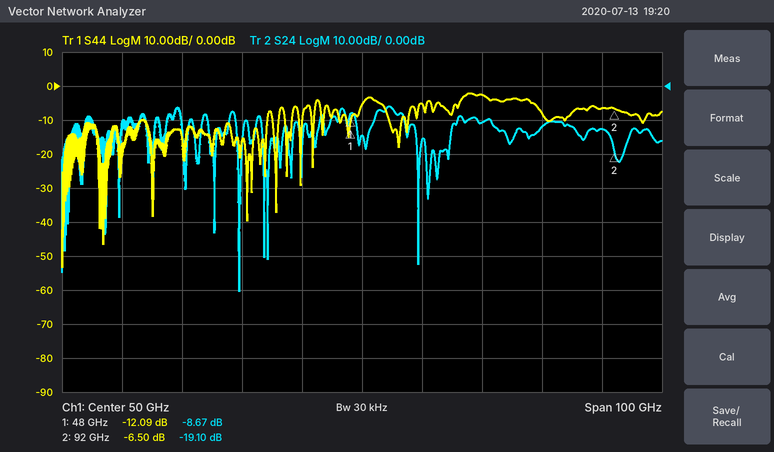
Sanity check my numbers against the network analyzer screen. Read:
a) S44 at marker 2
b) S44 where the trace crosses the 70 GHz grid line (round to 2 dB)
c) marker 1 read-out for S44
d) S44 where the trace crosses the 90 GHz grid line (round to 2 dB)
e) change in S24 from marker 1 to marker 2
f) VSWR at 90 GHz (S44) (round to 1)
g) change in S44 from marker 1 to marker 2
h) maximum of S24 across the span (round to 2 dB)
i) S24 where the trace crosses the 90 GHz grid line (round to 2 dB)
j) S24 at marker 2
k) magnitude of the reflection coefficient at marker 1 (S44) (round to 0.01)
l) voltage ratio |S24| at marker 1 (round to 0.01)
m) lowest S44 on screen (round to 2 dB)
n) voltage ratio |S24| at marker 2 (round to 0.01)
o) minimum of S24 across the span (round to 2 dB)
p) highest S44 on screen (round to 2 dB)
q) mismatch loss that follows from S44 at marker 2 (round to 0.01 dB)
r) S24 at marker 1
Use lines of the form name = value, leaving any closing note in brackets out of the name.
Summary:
S44 at marker 2 = -6.50 dB
S44 where the trace crosses the 70 GHz grid line = -2 dB
marker 1 read-out for S44 = -12.09 dB
S44 where the trace crosses the 90 GHz grid line = -6 dB
change in S24 from marker 1 to marker 2 = -10.43 dB
VSWR at 90 GHz (S44) = 3
change in S44 from marker 1 to marker 2 = 5.59 dB
maximum of S24 across the span = -6 dB
S24 where the trace crosses the 90 GHz grid line = -12 dB
S24 at marker 2 = -19.10 dB
magnitude of the reflection coefficient at marker 1 (S44) = 0.25
voltage ratio |S24| at marker 1 = 0.37
lowest S44 on screen = -54 dB
voltage ratio |S24| at marker 2 = 0.11
minimum of S24 across the span = -60 dB
highest S44 on screen = -2 dB
mismatch loss that follows from S44 at marker 2 = 1.10 dB
S24 at marker 1 = -8.67 dB
